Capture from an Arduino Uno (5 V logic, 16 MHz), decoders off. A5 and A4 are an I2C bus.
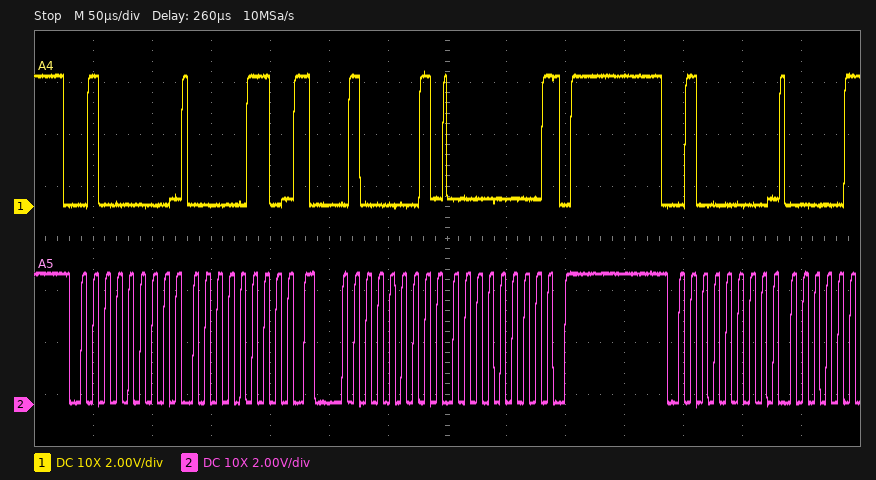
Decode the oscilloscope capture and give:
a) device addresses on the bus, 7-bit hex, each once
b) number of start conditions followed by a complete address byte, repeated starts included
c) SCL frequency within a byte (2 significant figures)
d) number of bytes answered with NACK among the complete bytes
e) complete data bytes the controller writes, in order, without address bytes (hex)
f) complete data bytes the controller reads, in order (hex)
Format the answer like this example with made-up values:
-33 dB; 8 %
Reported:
0x20; 3; 100 kHz; 1; 06; 00
